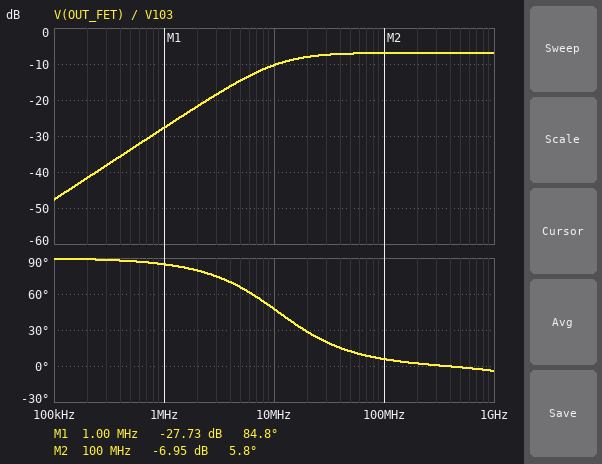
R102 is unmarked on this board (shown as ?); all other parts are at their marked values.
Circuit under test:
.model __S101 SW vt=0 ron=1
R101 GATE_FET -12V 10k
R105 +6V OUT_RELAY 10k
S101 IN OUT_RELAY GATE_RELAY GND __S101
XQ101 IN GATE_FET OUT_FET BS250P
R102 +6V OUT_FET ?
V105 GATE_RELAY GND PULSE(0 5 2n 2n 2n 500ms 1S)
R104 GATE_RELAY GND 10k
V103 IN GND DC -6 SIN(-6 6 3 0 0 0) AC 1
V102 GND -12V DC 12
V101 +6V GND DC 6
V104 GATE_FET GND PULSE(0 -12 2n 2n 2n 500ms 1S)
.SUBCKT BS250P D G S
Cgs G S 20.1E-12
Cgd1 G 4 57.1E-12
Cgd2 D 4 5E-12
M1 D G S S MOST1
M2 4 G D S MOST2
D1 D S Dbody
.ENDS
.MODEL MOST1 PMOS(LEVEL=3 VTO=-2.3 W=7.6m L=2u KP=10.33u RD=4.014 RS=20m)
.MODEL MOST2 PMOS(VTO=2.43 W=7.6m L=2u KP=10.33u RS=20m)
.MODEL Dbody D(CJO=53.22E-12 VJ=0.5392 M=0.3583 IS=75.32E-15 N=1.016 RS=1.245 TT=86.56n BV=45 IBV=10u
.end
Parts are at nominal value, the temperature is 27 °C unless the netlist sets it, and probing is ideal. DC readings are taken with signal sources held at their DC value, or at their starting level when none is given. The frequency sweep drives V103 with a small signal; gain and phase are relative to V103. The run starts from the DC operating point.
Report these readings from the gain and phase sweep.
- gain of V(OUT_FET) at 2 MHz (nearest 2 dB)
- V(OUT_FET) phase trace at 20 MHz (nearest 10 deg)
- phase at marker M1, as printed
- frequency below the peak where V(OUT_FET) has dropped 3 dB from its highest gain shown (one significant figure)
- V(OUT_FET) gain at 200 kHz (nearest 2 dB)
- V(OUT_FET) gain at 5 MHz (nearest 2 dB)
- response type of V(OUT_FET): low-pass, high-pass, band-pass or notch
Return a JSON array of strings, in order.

["-22 dB", "30 deg", "84.8 deg", "10 MHz", "-42 dB", "-14 dB", "high-pass"]
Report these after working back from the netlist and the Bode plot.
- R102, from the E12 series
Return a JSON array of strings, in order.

["33 kΩ"]
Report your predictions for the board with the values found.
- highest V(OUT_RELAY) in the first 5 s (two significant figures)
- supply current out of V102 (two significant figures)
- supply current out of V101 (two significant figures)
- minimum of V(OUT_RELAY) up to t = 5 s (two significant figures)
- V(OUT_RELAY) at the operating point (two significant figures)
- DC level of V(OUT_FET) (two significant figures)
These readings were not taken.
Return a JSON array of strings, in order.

["6.0 V", "1.2 mA", "1.3 mA", "-12 V", "-6.0 V", "2.4 V"]
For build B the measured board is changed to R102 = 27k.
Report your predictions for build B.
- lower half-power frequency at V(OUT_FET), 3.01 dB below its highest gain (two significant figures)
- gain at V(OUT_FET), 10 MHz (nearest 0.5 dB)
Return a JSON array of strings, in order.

["12 MHz", "-11.0 dB"]
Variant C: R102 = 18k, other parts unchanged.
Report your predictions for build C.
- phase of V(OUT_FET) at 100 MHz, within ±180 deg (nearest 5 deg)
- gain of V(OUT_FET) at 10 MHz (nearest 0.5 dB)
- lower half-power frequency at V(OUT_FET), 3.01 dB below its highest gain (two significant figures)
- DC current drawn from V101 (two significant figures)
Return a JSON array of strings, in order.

["10 deg", "-12.0 dB", "15 MHz", "1.4 mA"]
